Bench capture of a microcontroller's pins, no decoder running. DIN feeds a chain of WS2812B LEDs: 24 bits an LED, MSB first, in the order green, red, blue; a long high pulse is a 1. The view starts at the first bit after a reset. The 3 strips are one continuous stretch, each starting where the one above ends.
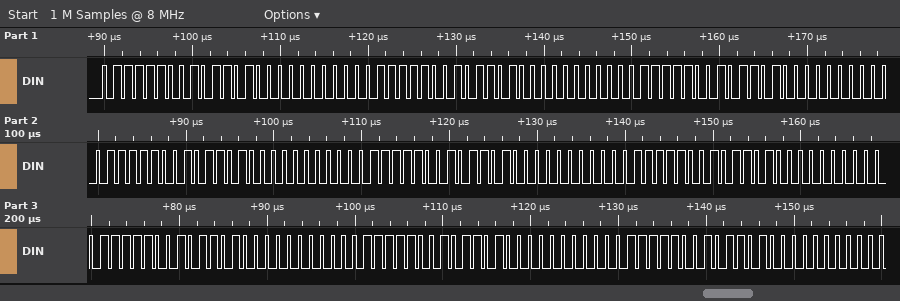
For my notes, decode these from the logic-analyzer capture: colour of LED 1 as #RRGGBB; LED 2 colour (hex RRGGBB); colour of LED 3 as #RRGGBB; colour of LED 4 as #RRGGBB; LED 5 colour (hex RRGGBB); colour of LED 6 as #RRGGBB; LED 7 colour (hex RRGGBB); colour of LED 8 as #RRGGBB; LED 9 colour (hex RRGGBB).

#B47C00
#B47C00
#B47C00
#B47C00
#B47C00
#B47C00
#B47C00
#B47C00
#B47C00
